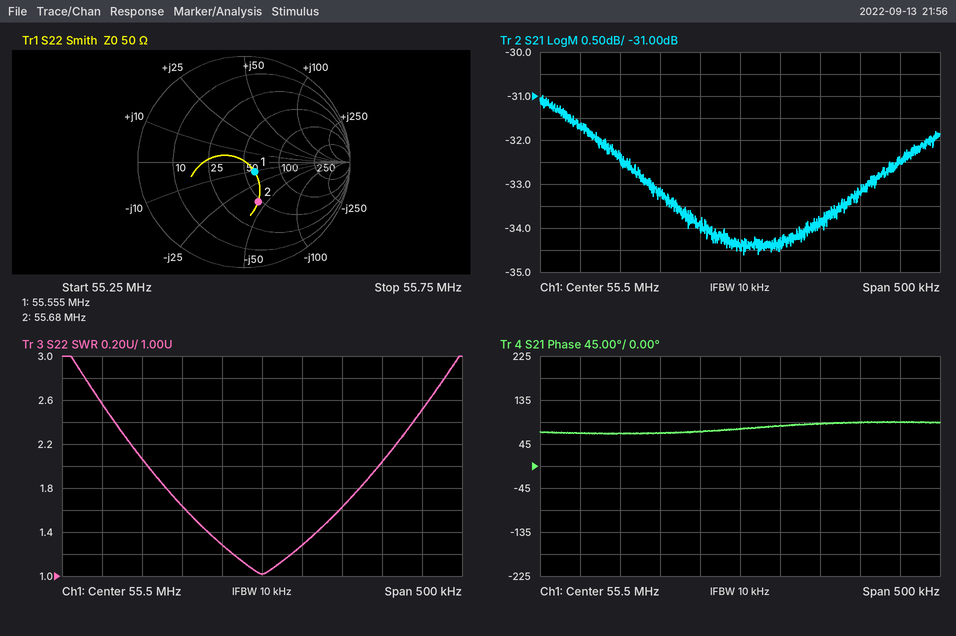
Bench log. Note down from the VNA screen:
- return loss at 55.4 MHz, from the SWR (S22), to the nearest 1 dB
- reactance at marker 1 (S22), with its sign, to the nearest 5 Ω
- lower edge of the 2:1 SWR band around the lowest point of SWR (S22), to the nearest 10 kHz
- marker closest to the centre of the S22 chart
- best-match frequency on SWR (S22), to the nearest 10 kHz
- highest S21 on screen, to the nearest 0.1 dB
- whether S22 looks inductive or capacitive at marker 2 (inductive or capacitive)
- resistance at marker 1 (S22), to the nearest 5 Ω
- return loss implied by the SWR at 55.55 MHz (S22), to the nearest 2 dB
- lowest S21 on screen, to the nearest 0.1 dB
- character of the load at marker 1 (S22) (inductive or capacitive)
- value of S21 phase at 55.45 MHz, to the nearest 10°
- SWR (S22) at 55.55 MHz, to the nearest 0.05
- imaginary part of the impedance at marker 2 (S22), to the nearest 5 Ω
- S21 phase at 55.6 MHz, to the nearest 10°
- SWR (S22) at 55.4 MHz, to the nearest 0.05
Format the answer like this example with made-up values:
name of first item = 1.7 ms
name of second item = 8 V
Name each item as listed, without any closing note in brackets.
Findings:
return loss at 55.4 MHz, from the SWR (S22), to the nearest 1 dB = 12 dB
reactance at marker 1 (S22), with its sign, to the nearest 5 Ω = -10 Ω
lower edge of the 2:1 SWR band around the lowest point of SWR (S22), to the nearest 10 kHz = 55.36 MHz
marker closest to the centre of the S22 chart = marker 1
best-match frequency on SWR (S22), to the nearest 10 kHz = 55.50 MHz
highest S21 on screen, to the nearest 0.1 dB = -31.0 dB
whether S22 looks inductive or capacitive at marker 2 = capacitive
resistance at marker 1 (S22), to the nearest 5 Ω = 60 Ω
return loss implied by the SWR at 55.55 MHz (S22), to the nearest 2 dB = 18 dB
lowest S21 on screen, to the nearest 0.1 dB = -34.6 dB
character of the load at marker 1 (S22) = capacitive
value of S21 phase at 55.45 MHz, to the nearest 10° = 70°
SWR (S22) at 55.55 MHz, to the nearest 0.05 = 1.30
imaginary part of the impedance at marker 2 (S22), to the nearest 5 Ω = -40 Ω
S21 phase at 55.6 MHz, to the nearest 10° = 90°
SWR (S22) at 55.4 MHz, to the nearest 0.05 = 1.65
